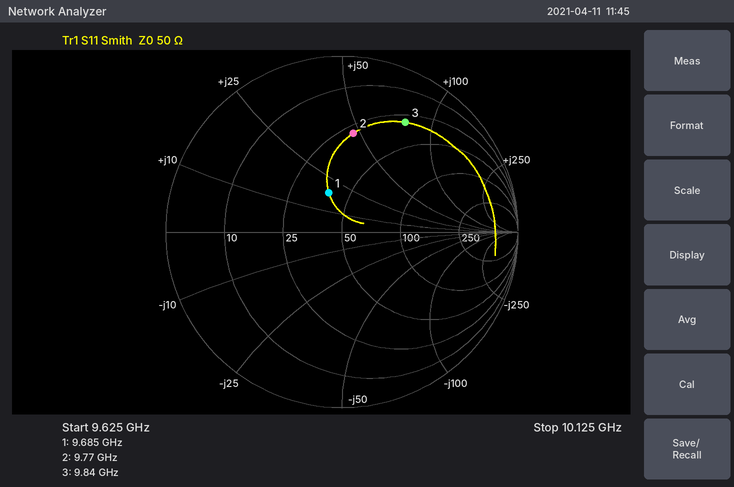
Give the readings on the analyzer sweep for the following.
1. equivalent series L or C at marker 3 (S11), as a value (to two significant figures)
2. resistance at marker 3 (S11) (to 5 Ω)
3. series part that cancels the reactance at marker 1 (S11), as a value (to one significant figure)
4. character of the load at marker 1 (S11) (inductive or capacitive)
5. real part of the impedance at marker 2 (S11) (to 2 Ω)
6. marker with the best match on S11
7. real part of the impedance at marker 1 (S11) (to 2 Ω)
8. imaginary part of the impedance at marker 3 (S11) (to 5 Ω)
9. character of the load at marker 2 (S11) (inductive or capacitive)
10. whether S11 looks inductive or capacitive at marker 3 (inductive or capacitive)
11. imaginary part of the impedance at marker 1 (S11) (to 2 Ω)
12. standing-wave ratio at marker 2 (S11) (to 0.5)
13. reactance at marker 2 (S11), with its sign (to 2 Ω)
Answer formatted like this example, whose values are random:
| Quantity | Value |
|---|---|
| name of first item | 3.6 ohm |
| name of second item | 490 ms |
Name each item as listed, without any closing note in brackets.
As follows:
| Quantity | Value |
|---|---|
| equivalent series L or C at marker 3 (S11), as a value | 1.3 nH |
| resistance at marker 3 (S11) | 30 Ω |
| series part that cancels the reactance at marker 1 (S11), as a value | 900 fF |
| character of the load at marker 1 (S11) | inductive |
| real part of the impedance at marker 2 (S11) | 28 Ω |
| marker with the best match on S11 | marker 1 |
| real part of the impedance at marker 1 (S11) | 40 Ω |
| imaginary part of the impedance at marker 3 (S11) | +80 Ω |
| character of the load at marker 2 (S11) | inductive |
| whether S11 looks inductive or capacitive at marker 3 | inductive |
| imaginary part of the impedance at marker 1 (S11) | +18 Ω |
| standing-wave ratio at marker 2 (S11) | 3.5 |
| reactance at marker 2 (S11), with its sign | +48 Ω |
